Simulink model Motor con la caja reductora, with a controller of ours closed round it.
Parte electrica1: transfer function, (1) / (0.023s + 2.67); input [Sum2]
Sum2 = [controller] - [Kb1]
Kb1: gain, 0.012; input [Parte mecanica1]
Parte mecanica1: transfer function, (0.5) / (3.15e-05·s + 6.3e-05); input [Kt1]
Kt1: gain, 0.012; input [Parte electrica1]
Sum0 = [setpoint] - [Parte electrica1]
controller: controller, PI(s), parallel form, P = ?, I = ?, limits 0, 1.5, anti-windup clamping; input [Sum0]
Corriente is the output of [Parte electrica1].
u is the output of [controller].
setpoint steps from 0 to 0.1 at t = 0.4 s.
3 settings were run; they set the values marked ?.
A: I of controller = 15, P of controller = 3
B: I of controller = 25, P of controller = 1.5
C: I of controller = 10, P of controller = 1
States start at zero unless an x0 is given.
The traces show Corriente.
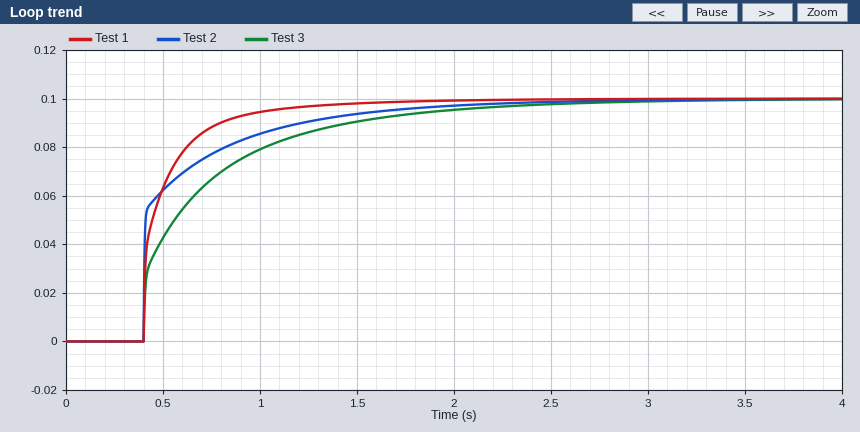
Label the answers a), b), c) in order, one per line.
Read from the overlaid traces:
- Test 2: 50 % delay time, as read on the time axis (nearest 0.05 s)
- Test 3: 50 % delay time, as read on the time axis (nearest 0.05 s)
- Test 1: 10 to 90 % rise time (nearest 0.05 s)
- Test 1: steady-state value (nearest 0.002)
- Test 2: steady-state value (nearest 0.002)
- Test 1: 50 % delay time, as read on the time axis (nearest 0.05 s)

a) 0.40 s
b) 0.55 s
c) 0.40 s
d) 0.100
e) 0.100
f) 0.45 s
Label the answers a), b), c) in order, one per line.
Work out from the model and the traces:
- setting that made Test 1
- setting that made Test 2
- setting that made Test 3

a) B
b) A
c) C
